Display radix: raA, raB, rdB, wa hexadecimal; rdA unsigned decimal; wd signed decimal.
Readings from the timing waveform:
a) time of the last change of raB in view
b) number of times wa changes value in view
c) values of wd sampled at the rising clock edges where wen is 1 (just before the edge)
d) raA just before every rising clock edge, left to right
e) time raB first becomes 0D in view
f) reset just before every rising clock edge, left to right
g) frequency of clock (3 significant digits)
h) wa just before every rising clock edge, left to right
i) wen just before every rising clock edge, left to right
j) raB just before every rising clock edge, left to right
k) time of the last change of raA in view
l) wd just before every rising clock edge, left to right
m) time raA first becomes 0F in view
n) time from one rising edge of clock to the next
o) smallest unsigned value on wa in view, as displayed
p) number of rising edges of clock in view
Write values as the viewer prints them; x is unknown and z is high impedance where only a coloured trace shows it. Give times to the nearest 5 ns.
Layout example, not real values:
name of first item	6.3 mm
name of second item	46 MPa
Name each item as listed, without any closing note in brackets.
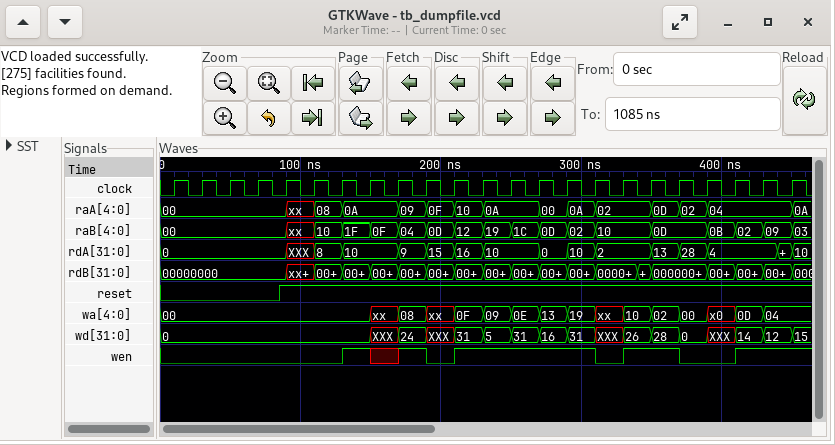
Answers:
time of the last change of raB in view	450 ns
number of times wa changes value in view	15
values of wd sampled at the rising clock edges where wen is 1	0, 24, 31, 5, 31, 16, 31, 26, 28, 14, 12
raA just before every rising clock edge, left to right	00, 00, 00, 00, 00, xx, 08, 0A, 0A, 09, 0F, 10, 0A, 0A, 00, 0A, 02, 02, 0D, 02, 04, 04, 04
time raB first becomes 0D in view	190 ns
reset just before every rising clock edge, left to right	0 0 0 0 1 1 1 1 1 1 1 1 1 1 1 1 1 1 1 1 1 1 1
frequency of clock	50.0 MHz
wa just before every rising clock edge, left to right	00, 00, 00, 00, 00, 00, 00, 00, xx, 08, xx, 0F, 09, 0E, 13, 19, xx, 10, 02, 00, x0, 0D, 04
wen just before every rising clock edge, left to right	0 0 0 0 0 0 0 1 x 1 0 1 1 1 1 1 0 1 1 0 0 1 1
raB just before every rising clock edge, left to right	00, 00, 00, 00, 00, xx, 10, 1F, 0F, 04, 0D, 12, 19, 1C, 0D, 02, 10, 10, 0D, 0D, 0B, 02, 09
time of the last change of raA in view	450 ns
wd just before every rising clock edge, left to right	0, 0, 0, 0, 0, 0, 0, 0, XXX, 24, XXX, 31, 5, 31, 16, 31, XXX, 26, 28, 0, XXX, 14, 12
time raA first becomes 0F in view	190 ns
time from one rising edge of clock to the next	20 ns
smallest unsigned value on wa in view, as displayed	00
number of rising edges of clock in view	23
